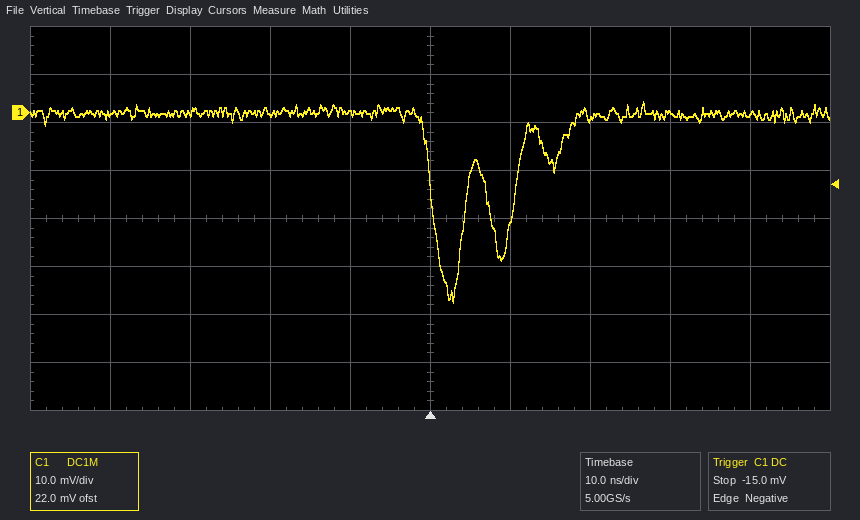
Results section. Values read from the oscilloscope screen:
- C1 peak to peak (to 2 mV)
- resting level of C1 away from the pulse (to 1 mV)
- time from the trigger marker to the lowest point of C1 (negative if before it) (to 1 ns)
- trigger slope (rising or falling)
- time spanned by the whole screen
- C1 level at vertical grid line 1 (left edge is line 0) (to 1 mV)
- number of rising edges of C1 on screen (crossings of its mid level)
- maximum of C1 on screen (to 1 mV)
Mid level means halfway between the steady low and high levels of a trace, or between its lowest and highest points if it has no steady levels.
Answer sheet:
42 mV
0 mV
+3 ns
falling
100 ns
0 mV
2
2 mV
